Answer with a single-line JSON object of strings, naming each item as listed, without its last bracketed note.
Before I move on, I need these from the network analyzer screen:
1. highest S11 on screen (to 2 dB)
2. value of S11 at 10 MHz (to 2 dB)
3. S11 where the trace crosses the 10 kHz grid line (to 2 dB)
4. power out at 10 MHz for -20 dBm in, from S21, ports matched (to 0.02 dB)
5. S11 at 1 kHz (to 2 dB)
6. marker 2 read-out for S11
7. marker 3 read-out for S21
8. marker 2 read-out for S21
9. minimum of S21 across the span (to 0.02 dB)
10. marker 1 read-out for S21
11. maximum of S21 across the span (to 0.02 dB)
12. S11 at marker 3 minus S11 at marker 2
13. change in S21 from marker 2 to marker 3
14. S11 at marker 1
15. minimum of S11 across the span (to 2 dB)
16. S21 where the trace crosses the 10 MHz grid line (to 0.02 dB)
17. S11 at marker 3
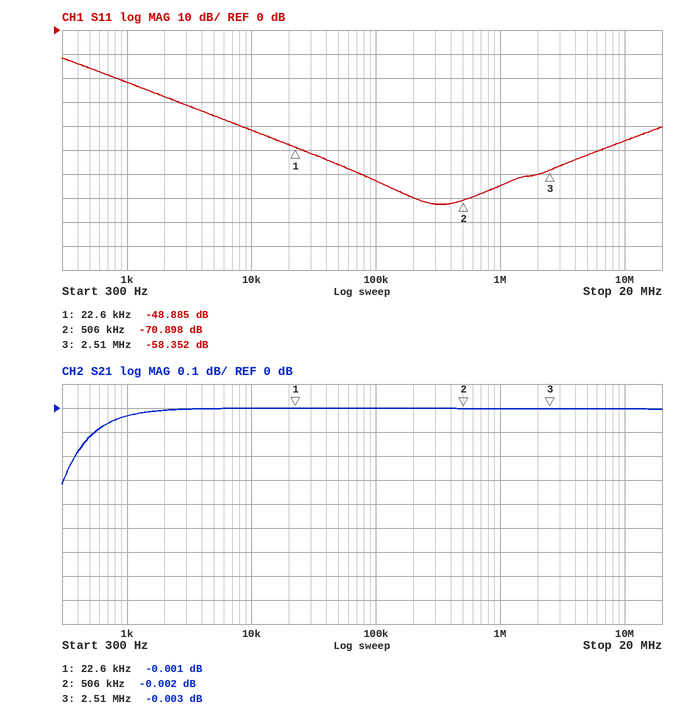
{"highest S11 on screen": "-12 dB", "value of S11 at 10 MHz": "-46 dB", "S11 where the trace crosses the 10 kHz grid line": "-42 dB", "power out at 10 MHz for -20 dBm in, from S21, ports matched": "-20.00 dBm", "S11 at 1 kHz": "-22 dB", "marker 2 read-out for S11": "-70.898 dB", "marker 3 read-out for S21": "-0.003 dB", "marker 2 read-out for S21": "-0.002 dB", "minimum of S21 across the span": "-0.32 dB", "marker 1 read-out for S21": "-0.001 dB", "maximum of S21 across the span": "0.00 dB", "S11 at marker 3 minus S11 at marker 2": "12.546 dB", "change in S21 from marker 2 to marker 3": "-0.001 dB", "S11 at marker 1": "-48.885 dB", "minimum of S11 across the span": "-72 dB", "S21 where the trace crosses the 10 MHz grid line": "0.00 dB", "S11 at marker 3": "-58.352 dB"}
